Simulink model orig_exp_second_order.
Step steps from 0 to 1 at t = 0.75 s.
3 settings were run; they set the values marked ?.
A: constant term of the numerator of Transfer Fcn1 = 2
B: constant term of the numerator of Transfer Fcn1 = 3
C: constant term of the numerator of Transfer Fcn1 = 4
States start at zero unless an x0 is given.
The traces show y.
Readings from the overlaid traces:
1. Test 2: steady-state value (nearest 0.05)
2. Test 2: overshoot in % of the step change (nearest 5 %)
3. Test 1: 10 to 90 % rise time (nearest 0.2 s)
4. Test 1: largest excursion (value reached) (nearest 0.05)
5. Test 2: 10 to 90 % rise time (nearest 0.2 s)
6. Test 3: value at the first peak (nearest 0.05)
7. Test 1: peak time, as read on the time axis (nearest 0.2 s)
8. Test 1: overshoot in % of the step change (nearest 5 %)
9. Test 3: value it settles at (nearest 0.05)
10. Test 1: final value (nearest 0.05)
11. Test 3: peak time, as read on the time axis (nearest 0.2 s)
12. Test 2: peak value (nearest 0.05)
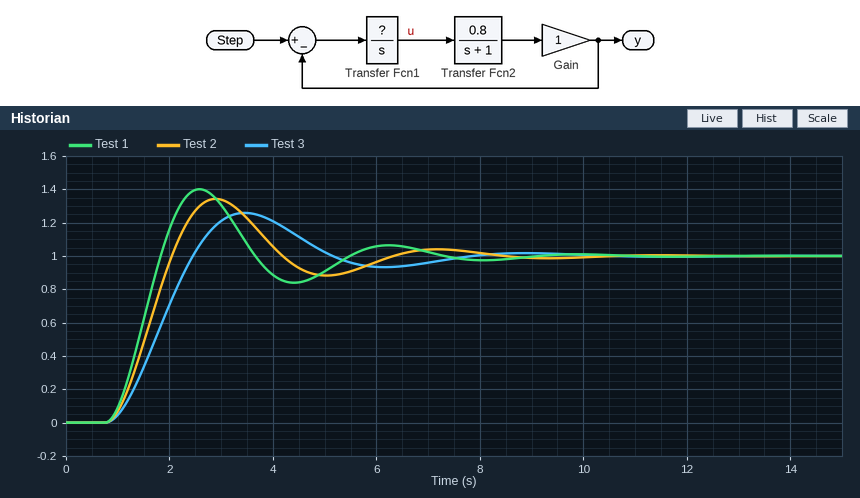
1.00
35 %
0.8 s
1.40
0.8 s
1.25
2.6 s
40 %
1.00
1.00
3.4 s
1.35
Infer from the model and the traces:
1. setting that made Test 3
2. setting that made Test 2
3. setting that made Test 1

A
B
C
